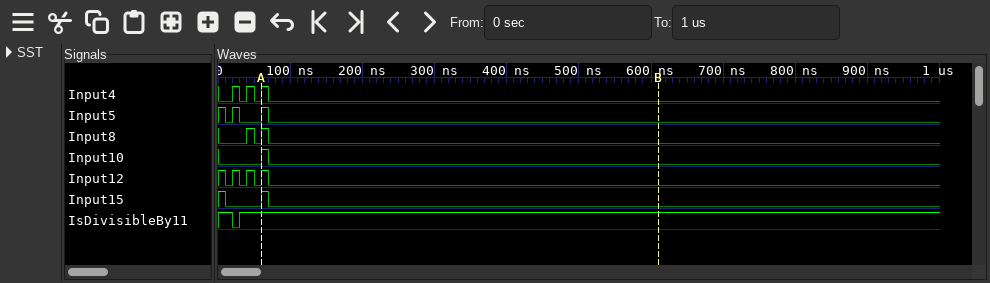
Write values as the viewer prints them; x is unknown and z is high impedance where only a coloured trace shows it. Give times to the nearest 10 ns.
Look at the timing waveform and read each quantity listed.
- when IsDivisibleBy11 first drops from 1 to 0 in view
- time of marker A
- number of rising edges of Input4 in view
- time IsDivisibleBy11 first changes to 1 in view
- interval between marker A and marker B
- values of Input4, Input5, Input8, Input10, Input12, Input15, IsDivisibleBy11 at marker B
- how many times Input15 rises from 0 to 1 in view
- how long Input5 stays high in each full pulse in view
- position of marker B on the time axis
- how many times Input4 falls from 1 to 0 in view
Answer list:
20 ns
60 ns
3
30 ns
550 ns
Input4=0, Input5=0, Input8=0, Input10=0, Input12=0, Input15=0, IsDivisibleBy11=1
1
10 ns, 10 ns
610 ns
3
